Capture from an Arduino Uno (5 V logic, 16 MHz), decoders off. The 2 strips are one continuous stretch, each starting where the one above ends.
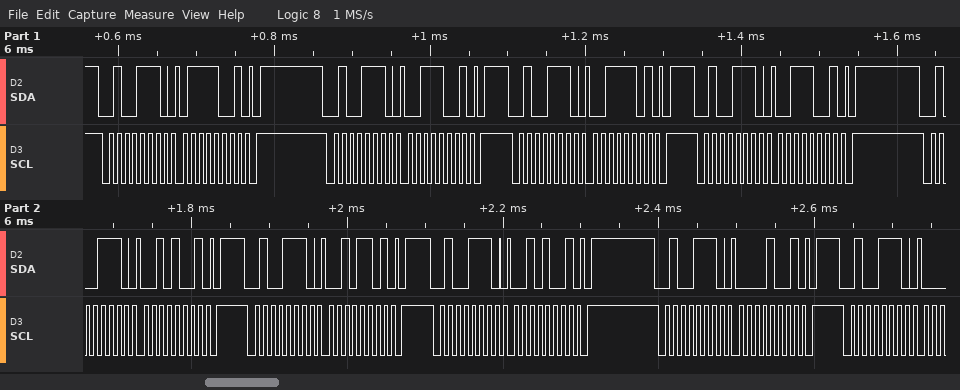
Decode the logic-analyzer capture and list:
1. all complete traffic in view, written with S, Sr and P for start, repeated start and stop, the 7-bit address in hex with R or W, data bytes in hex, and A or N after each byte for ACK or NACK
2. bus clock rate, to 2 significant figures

S 27W A 79 A P S 27W A 39 A P S 27W A 3D A P S 27W A 39 A P S 27W A 29 A P S 27W A 2D A P S 27W A 29 A P S 27W A 09 A P S 27W A
100 kHz
